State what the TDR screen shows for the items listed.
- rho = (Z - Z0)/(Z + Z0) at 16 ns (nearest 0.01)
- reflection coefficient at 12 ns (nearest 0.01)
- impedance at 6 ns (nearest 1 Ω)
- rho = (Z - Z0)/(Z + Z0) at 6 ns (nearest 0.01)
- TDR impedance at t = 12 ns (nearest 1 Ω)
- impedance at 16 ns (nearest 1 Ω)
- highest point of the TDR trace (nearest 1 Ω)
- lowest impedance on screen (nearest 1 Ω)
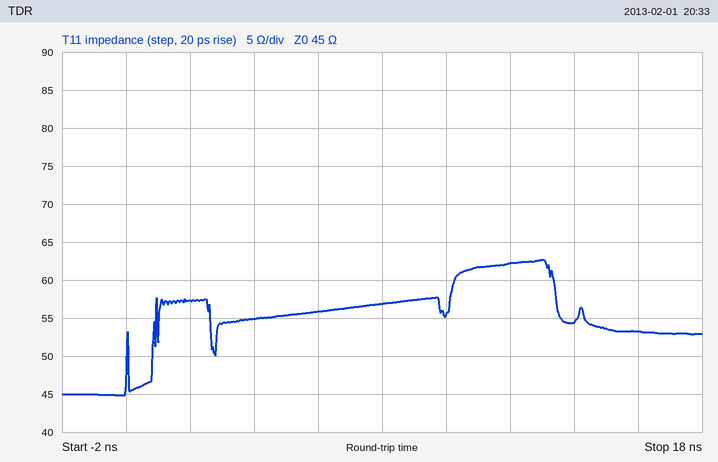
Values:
+0.08
+0.16
56 Ω
+0.11
62 Ω
53 Ω
63 Ω
45 Ω
